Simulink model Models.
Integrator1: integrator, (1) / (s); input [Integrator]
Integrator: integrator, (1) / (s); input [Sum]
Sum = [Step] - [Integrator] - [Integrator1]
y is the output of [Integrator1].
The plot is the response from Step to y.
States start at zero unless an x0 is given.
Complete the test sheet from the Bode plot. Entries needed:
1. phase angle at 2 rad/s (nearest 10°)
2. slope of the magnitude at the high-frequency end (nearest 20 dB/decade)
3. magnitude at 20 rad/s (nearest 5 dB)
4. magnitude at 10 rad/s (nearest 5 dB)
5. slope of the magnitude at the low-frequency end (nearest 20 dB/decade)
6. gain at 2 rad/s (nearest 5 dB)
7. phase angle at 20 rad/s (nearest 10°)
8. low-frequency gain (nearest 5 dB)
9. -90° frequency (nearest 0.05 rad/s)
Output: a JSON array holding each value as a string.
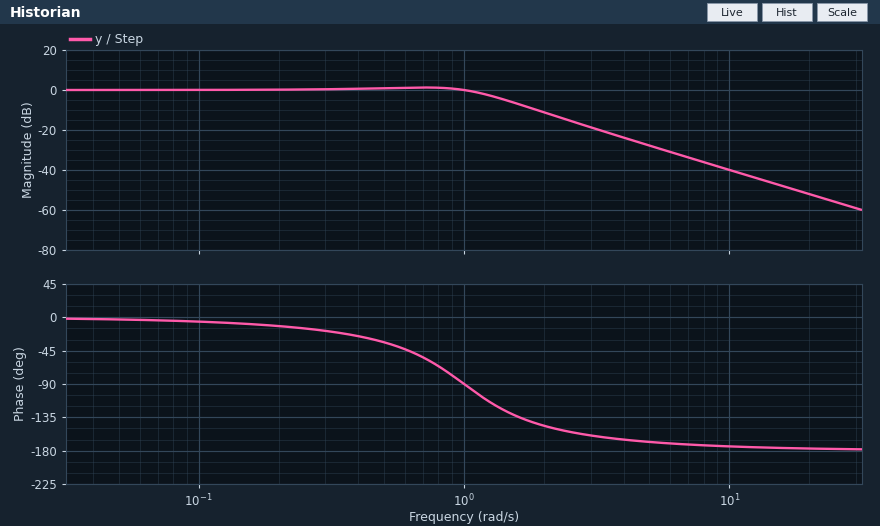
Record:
["-150°", "-40 dB/decade", "-50 dB", "-40 dB", "0 dB/decade", "-10 dB", "-180°", "0 dB", "1.00 rad/s"]
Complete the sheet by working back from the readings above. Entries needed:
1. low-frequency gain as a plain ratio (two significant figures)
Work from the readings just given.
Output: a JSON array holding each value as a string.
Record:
["1.0"]
